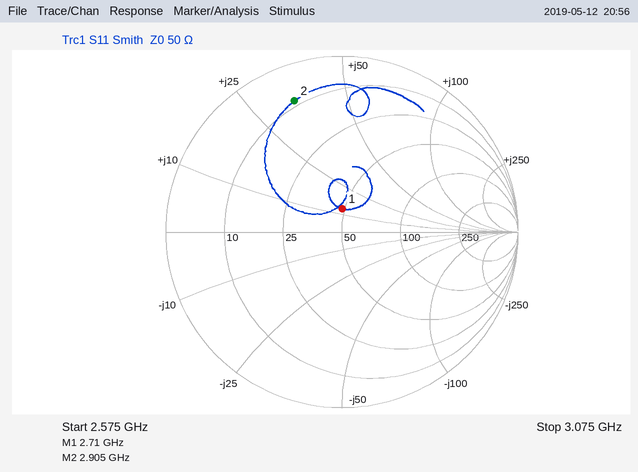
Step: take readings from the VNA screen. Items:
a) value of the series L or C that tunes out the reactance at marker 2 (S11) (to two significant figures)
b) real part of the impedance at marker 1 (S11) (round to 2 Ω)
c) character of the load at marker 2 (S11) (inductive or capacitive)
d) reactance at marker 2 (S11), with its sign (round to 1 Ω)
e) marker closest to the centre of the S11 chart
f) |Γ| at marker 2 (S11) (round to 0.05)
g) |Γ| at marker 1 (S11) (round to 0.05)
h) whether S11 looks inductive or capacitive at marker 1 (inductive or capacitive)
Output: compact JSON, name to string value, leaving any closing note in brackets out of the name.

{"value of the series L or C that tunes out the reactance at marker 2 (S11)": "1.6 pF", "real part of the impedance at marker 1 (S11)": "48 Ω", "character of the load at marker 2 (S11)": "inductive", "reactance at marker 2 (S11), with its sign": "+34 Ω", "marker closest to the centre of the S11 chart": "marker 1", "|Γ| at marker 2 (S11)": "0.80", "|Γ| at marker 1 (S11)": "0.15", "whether S11 looks inductive or capacitive at marker 1": "inductive"}
